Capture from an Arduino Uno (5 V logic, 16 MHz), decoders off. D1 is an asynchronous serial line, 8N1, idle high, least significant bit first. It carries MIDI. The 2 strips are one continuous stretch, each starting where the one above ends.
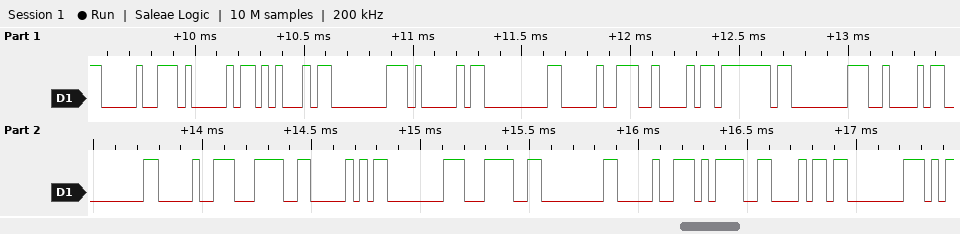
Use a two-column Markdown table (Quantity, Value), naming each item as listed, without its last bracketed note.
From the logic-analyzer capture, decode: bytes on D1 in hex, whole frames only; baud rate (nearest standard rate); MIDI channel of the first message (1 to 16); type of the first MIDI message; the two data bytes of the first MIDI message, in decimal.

| Quantity | Value |
|---|---|
| bytes on D1 in hex, whole frames only | 90 41 45 80 41 00 90 42 7F 80 42 00 90 3C 50 80 3C 00 90 3D 68 80 |
| baud rate | 31250 baud |
| MIDI channel of the first message | 1 |
| type of the first MIDI message | Note On |
| the two data bytes of the first MIDI message, in decimal | 65, 69 |
